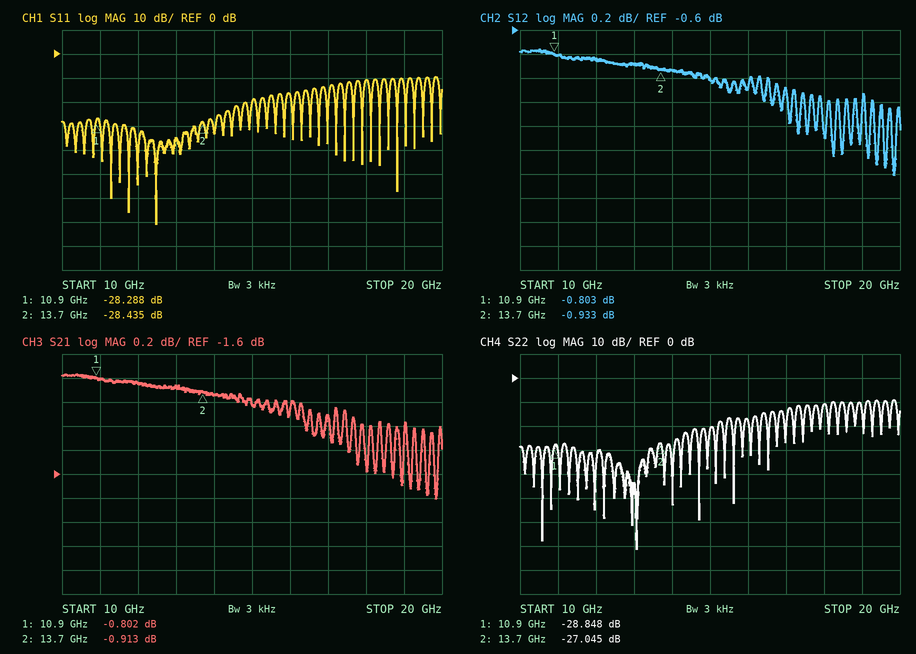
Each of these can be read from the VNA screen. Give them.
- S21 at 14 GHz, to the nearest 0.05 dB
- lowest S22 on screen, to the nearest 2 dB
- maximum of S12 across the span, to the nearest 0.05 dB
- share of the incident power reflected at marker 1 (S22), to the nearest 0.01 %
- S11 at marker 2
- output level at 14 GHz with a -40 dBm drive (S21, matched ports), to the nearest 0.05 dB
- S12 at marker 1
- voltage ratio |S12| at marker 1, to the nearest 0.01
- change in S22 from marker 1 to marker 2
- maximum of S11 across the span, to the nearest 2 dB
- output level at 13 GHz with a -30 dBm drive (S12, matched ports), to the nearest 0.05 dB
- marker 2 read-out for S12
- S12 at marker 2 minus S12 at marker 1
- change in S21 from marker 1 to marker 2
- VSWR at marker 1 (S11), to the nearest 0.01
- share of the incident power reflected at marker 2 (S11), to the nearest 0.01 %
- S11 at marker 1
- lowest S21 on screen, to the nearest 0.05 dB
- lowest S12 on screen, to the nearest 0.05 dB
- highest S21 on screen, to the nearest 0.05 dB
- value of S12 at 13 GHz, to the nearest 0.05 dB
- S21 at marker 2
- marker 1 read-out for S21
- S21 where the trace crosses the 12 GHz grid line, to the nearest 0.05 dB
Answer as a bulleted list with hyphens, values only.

- -0.95 dB
- -72 dB
- -0.75 dB
- 0.13 %
- -28.435 dB
- -40.95 dBm
- -0.803 dB
- 0.91
- 1.803 dB
- -10 dB
- -30.90 dBm
- -0.933 dB
- -0.130 dB
- -0.111 dB
- 1.08
- 0.14 %
- -28.288 dB
- -1.80 dB
- -1.80 dB
- -0.75 dB
- -0.90 dB
- -0.913 dB
- -0.802 dB
- -0.85 dB
